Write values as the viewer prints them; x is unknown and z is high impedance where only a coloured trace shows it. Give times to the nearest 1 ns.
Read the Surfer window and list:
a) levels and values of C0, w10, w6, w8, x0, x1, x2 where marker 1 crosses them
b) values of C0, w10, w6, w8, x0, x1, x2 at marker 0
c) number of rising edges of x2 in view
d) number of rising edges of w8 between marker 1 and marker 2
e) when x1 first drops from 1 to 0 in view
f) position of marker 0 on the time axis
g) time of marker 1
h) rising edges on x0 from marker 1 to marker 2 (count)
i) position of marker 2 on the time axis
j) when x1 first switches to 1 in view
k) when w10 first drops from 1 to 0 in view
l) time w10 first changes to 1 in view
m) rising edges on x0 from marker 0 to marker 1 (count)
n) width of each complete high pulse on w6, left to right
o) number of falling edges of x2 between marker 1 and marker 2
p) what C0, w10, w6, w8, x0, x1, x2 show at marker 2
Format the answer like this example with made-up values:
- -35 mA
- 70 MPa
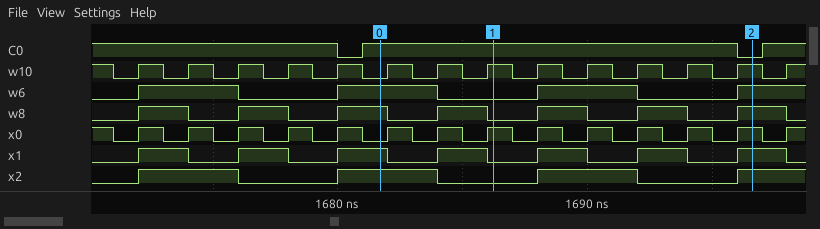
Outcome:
- C0=1, w10=1, w6=0, w8=0, x0=1, x1=0, x2=0
- C0=1, w10=0, w6=1, w8=1, x0=0, x1=1, x2=1
- 4
- 3
- 1674 ns
- 1682 ns
- 1686 ns
- 5
- 1697 ns
- 1672 ns
- 1671 ns
- 1672 ns
- 3
- 4 ns, 4 ns, 4 ns
- 1
- C0=0, w10=1, w6=1, w8=1, x0=1, x1=1, x2=1
